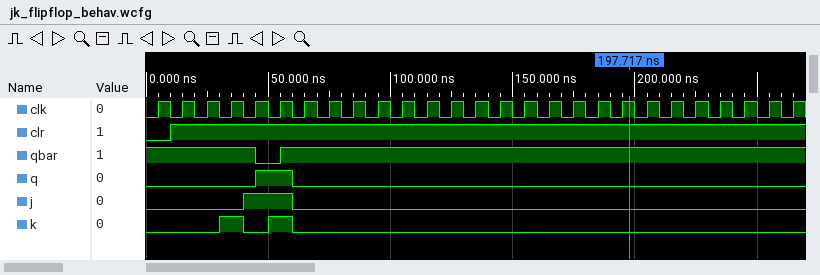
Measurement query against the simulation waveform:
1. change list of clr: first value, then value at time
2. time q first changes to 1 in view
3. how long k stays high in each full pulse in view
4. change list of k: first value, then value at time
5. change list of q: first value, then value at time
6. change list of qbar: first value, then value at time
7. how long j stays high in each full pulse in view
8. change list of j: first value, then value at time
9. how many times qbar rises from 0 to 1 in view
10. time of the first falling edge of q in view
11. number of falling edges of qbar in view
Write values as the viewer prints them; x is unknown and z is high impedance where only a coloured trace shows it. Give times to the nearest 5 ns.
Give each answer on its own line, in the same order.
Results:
0, 1 at 10 ns
45 ns
10 ns, 10 ns
0, 1 at 30 ns, 0 at 40 ns, 1 at 50 ns, 0 at 60 ns
0, 1 at 45 ns, 0 at 60 ns
1, 0 at 45 ns, 1 at 55 ns
20 ns
0, 1 at 40 ns, 0 at 60 ns
1
60 ns
1
